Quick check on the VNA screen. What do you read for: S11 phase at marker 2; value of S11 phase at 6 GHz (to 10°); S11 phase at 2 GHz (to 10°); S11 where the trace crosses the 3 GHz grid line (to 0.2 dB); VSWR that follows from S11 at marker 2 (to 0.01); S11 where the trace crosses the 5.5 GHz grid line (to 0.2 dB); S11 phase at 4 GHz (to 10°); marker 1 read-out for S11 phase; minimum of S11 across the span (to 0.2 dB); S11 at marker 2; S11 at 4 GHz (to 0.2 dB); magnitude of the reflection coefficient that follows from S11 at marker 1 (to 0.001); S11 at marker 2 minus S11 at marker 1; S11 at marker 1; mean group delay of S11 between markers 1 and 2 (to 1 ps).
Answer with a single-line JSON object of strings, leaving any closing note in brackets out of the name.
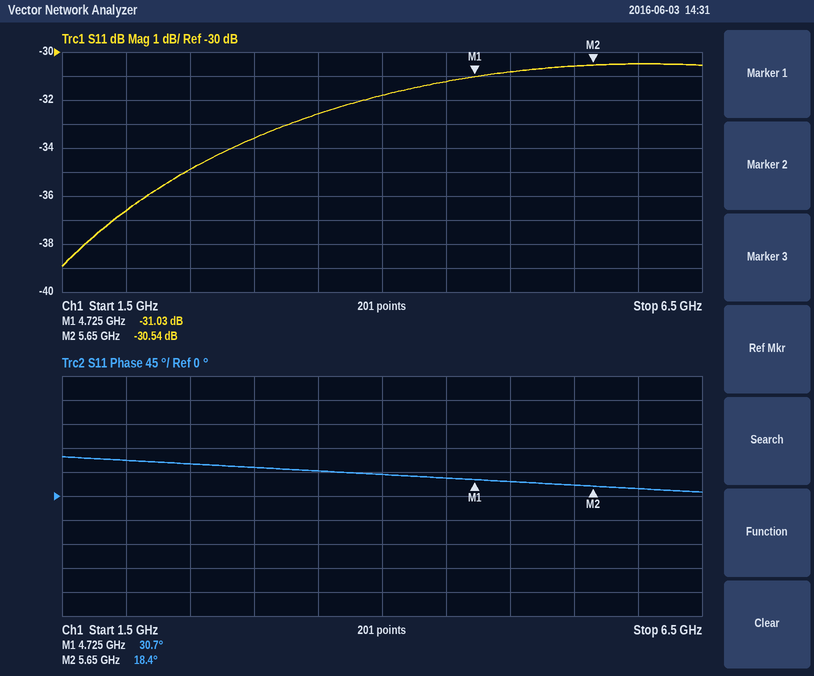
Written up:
{"S11 phase at marker 2": "18.4°", "value of S11 phase at 6 GHz": "10°", "S11 phase at 2 GHz": "70°", "S11 where the trace crosses the 3 GHz grid line": "-33.6 dB", "VSWR that follows from S11 at marker 2": "1.06", "S11 where the trace crosses the 5.5 GHz grid line": "-30.6 dB", "S11 phase at 4 GHz": "40°", "marker 1 read-out for S11 phase": "30.7°", "minimum of S11 across the span": "-39.0 dB", "S11 at marker 2": "-30.54 dB", "S11 at 4 GHz": "-31.8 dB", "magnitude of the reflection coefficient that follows from S11 at marker 1": "0.028", "S11 at marker 2 minus S11 at marker 1": "0.49 dB", "S11 at marker 1": "-31.03 dB", "mean group delay of S11 between markers 1 and 2": "37 ps"}
